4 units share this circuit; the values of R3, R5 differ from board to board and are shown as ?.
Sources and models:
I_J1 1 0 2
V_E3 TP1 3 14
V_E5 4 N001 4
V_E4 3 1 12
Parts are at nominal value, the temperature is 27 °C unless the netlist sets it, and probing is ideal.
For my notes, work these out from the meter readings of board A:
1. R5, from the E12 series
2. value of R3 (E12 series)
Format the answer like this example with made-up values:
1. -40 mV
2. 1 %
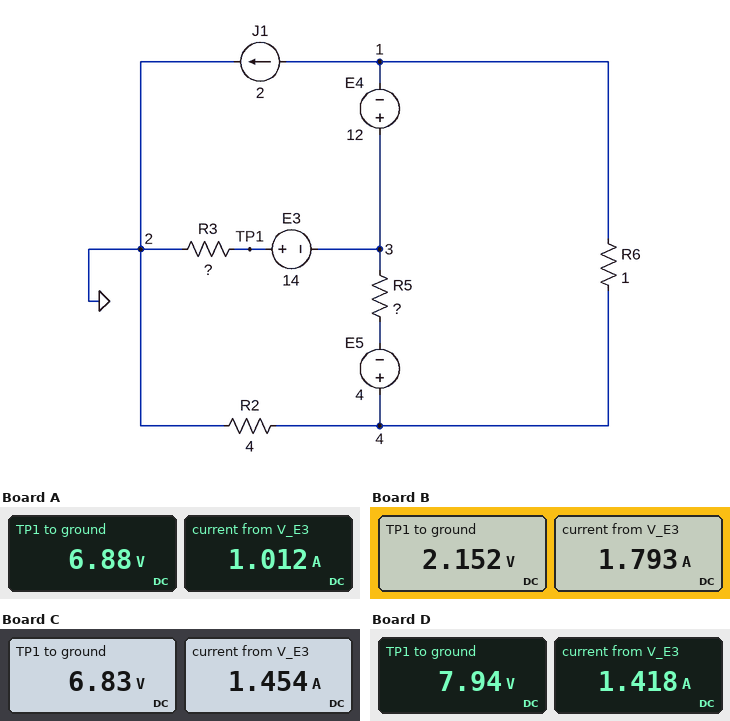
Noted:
1. 2.2 Ω
2. 6.8 Ω
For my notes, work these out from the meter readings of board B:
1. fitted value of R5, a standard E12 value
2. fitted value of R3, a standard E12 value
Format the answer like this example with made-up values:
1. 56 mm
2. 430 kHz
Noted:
1. 1.5 Ω
2. 1.2 Ω
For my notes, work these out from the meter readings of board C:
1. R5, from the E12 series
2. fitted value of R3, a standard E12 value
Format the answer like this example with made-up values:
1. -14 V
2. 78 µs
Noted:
1. 5.6 Ω
2. 4.7 Ω
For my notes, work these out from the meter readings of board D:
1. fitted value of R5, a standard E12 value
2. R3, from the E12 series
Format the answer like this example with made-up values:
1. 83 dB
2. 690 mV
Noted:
1. 12 Ω
2. 5.6 Ω
